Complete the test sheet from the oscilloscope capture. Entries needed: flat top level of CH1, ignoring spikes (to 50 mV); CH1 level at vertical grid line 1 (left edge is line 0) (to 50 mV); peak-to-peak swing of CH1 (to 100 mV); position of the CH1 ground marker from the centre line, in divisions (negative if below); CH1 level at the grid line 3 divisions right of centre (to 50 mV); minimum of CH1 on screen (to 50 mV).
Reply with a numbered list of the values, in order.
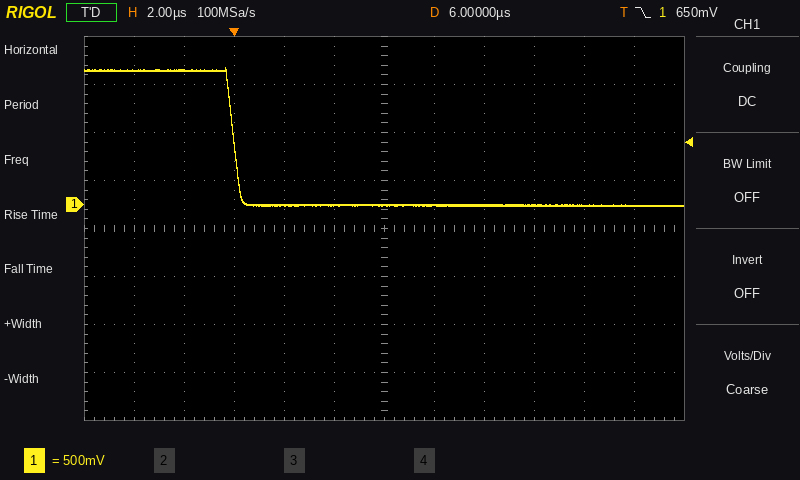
1. 1.40 V
2. 1.40 V
3. 1.40 V
4. +0.5 div
5. 0 mV
6. 0 mV
